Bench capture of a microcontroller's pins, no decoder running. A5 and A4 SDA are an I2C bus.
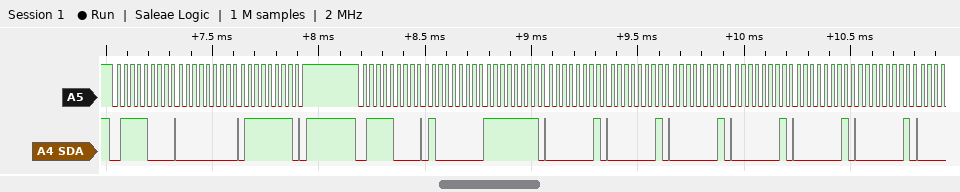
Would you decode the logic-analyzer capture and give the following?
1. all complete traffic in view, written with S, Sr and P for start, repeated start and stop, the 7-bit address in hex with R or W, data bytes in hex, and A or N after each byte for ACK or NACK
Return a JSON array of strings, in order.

["S 3CW A 00 A 7F A P S 3CW A 40 A FF A 01 A 01 A 01 A 01 A 01 A 01 A"]
